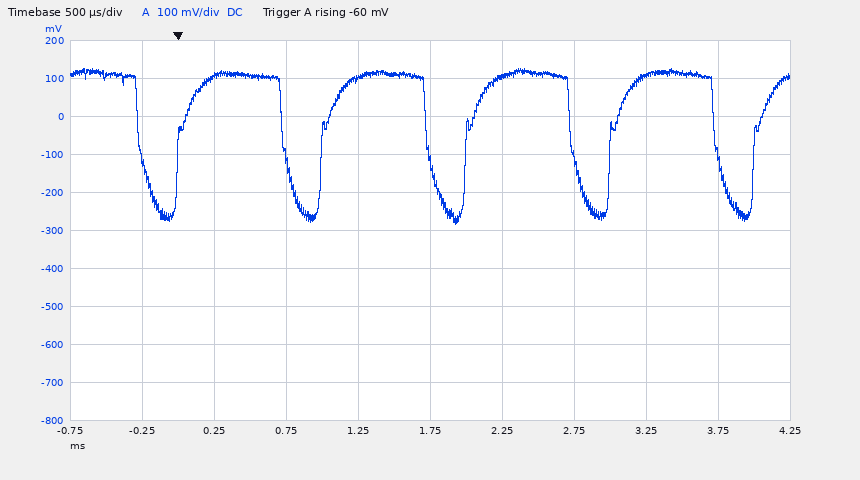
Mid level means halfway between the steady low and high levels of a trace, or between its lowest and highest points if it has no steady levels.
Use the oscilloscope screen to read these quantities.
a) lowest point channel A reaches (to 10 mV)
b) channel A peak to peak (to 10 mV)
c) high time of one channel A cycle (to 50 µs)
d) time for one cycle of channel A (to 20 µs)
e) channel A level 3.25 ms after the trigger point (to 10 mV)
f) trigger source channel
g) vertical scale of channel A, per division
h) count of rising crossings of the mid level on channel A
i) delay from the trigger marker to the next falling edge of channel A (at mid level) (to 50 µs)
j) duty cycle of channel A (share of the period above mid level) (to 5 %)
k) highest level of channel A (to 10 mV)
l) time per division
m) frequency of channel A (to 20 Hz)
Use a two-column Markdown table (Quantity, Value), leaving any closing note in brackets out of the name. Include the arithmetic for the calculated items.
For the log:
| Quantity | Value |
|---|---|
| lowest point channel A reaches | -280 mV |
| channel A peak to peak | 130 mV − (-280 mV) = 410 mV |
| high time of one channel A cycle | 750 µs |
| time for one cycle of channel A | 1.00 ms |
| channel A level 3.25 ms after the trigger point | 110 mV |
| trigger source channel | channel A |
| vertical scale of channel A, per division | 100 mV |
| count of rising crossings of the mid level on channel A | 5 |
| delay from the trigger marker to the next falling edge of channel A (at mid level) | 750 µs |
| duty cycle of channel A (share of the period above mid level) | 750 µs / 1.00 ms ≈ 75 % |
| highest level of channel A | 130 mV |
| time per division | 500 µs |
| frequency of channel A | 1 / 1.00 ms ≈ 1.00 kHz |
